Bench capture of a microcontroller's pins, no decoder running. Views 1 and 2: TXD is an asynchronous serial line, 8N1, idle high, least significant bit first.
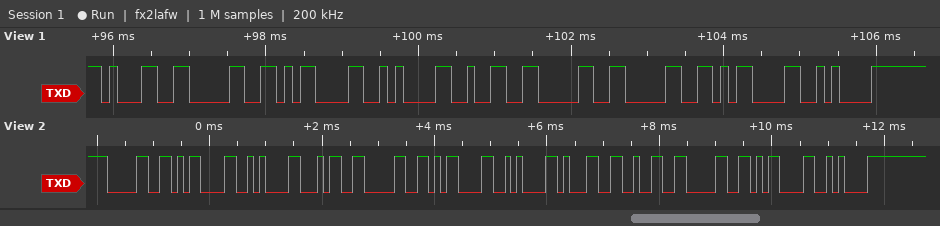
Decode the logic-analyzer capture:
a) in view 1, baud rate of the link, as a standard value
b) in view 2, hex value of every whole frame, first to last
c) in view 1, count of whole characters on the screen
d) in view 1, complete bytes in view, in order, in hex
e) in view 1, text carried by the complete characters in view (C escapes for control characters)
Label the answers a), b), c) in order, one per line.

a) 9600 baud
b) 30 0D 0A 34 30 0D 0A 31 32 30 0D 0A
c) 9
d) 31 30 0D 0A 32 30 30 0D 0A
e) "10\r\n200\r\n"
